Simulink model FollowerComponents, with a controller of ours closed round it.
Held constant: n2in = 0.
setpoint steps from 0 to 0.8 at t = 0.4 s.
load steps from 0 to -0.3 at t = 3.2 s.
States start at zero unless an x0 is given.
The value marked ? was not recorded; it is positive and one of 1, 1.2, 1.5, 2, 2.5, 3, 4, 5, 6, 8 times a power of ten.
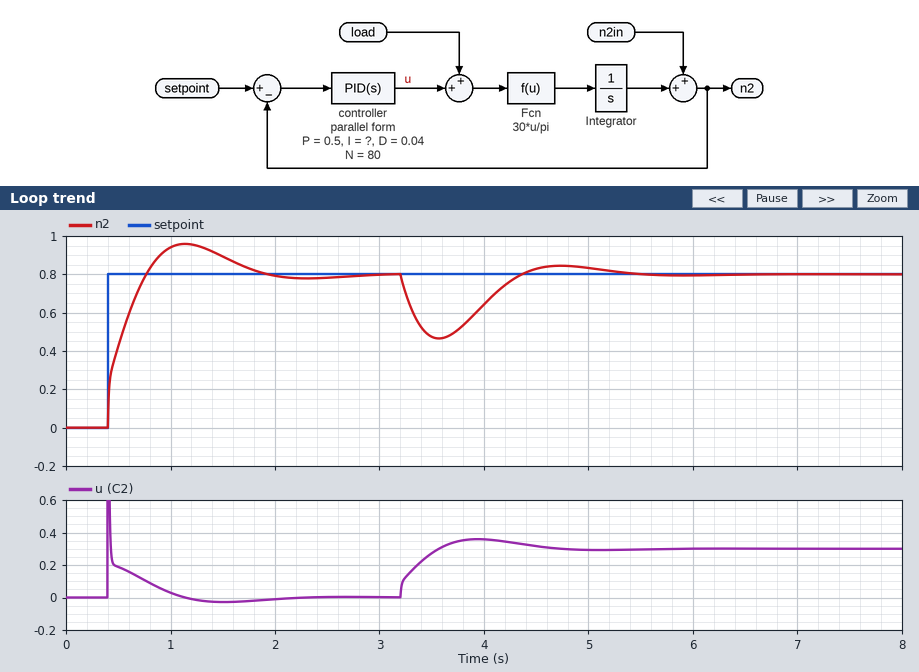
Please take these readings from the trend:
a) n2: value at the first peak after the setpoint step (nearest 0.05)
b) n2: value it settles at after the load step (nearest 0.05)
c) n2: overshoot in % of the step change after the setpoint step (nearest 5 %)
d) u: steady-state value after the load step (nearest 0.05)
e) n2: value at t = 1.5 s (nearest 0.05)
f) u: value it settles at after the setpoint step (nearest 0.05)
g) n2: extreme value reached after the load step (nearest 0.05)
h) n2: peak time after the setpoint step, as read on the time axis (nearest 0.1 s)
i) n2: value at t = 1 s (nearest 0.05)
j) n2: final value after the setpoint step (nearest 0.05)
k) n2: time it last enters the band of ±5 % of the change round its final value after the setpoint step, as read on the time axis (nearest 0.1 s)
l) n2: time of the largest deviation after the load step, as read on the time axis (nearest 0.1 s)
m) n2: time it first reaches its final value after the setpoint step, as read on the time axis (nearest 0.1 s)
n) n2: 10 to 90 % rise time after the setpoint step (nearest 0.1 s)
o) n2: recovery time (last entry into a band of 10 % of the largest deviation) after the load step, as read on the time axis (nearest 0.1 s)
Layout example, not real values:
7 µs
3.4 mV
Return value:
0.95
0.80
20 %
0.30
0.90
0.00
0.45
1.1 s
0.95
0.80
1.7 s
3.6 s
0.8 s
0.3 s
5.0 s
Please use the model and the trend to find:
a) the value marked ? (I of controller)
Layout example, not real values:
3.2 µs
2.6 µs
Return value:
1.5
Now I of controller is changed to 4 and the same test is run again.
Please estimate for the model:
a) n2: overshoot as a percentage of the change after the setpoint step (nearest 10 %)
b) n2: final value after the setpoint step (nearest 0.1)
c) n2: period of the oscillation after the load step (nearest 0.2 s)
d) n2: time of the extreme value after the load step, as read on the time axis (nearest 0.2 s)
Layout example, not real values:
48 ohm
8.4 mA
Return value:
30 %
0.8
1.2 s
3.4 s
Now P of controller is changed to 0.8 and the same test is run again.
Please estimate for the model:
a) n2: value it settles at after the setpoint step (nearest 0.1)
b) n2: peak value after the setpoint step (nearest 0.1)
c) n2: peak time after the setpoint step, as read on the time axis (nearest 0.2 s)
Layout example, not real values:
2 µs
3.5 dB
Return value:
0.8
0.9
1.0 s
